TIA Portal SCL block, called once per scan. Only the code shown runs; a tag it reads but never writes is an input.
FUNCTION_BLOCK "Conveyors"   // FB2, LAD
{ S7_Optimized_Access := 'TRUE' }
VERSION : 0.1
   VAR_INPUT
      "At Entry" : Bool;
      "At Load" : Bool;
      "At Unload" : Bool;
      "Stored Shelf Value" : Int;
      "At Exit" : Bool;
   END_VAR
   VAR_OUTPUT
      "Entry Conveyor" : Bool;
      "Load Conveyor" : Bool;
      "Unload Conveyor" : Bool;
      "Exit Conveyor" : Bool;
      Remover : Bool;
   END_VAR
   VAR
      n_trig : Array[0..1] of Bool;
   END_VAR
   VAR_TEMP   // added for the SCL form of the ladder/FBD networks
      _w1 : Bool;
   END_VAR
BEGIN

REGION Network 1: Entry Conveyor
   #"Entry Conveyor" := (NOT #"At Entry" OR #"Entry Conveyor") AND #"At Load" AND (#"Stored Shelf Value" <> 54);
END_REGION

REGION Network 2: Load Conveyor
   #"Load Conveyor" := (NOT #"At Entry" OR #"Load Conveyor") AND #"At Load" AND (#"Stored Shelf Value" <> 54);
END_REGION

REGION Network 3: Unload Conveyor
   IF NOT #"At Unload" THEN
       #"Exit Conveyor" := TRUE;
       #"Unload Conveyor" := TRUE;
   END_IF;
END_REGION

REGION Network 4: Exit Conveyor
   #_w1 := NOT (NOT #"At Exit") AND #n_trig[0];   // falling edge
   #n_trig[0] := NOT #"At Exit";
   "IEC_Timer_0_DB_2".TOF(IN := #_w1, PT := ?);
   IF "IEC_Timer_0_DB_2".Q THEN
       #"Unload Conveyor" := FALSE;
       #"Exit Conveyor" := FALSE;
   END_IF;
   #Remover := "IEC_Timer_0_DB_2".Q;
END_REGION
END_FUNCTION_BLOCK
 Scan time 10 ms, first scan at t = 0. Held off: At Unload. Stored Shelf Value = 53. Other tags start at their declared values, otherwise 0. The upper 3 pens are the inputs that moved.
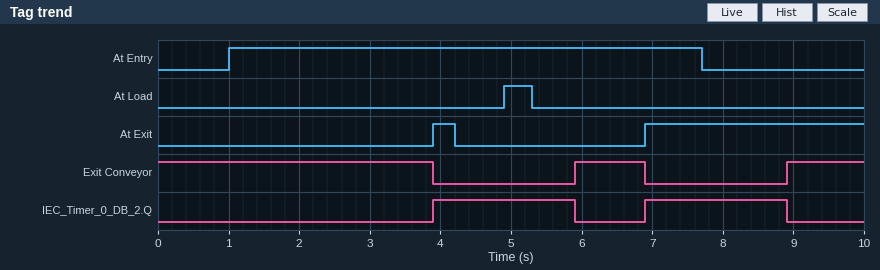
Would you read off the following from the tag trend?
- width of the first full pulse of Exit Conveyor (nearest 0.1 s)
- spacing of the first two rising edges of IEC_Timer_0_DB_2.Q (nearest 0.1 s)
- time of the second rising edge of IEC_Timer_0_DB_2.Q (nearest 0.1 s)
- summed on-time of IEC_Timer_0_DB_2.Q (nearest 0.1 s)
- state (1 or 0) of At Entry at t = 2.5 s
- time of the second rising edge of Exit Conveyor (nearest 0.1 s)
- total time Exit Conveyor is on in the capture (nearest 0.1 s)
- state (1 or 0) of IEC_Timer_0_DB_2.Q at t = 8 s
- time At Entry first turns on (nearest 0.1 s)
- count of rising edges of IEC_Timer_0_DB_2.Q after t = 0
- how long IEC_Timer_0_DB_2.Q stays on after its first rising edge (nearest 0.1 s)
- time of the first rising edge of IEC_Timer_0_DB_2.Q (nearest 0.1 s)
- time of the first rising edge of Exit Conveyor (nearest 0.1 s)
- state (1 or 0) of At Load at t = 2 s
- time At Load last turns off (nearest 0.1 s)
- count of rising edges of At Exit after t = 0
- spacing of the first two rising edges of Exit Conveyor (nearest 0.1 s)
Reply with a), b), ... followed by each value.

a) 1.0 s
b) 3.0 s
c) 6.9 s
d) 4.0 s
e) 1
f) 8.9 s
g) 6.0 s
h) 1
i) 1.0 s
j) 2
k) 2.0 s
l) 3.9 s
m) 5.9 s
n) 0
o) 5.3 s
p) 2
q) 3.0 s
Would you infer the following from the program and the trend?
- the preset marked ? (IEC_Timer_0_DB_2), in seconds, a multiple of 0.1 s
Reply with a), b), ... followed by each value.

a) 2.0 s
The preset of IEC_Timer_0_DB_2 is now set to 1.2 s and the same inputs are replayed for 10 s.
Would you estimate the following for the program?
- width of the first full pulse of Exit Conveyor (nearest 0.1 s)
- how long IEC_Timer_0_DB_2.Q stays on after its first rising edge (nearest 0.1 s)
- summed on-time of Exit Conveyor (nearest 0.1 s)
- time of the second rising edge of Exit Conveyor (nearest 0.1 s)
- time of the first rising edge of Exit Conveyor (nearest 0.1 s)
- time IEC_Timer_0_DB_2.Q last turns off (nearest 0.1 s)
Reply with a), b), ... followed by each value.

a) 1.8 s
b) 1.2 s
c) 7.6 s
d) 8.1 s
e) 5.1 s
f) 8.1 s
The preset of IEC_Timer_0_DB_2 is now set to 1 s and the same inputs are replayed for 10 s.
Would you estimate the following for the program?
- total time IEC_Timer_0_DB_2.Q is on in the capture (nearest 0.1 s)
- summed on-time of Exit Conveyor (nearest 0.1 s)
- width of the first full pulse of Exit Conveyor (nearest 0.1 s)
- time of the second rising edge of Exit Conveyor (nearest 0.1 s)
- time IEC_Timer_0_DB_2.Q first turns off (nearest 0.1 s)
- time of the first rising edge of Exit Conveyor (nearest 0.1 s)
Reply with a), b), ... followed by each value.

a) 2.0 s
b) 8.0 s
c) 2.0 s
d) 7.9 s
e) 4.9 s
f) 4.9 s
